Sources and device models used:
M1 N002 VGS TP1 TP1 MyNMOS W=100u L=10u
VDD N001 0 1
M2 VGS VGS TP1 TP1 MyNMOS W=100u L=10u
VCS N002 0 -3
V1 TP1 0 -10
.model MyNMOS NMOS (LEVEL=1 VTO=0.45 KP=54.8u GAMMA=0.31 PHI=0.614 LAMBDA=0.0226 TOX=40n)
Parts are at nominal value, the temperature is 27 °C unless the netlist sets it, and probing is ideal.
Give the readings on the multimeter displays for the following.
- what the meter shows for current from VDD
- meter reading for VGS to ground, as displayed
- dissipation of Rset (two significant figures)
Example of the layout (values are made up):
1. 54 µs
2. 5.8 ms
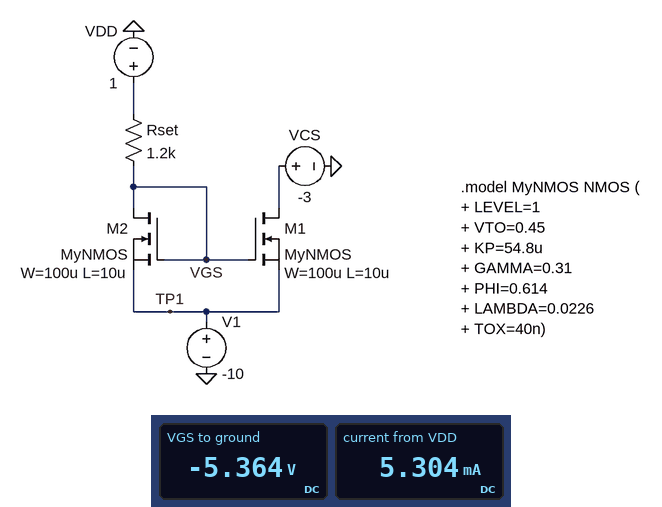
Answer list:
1. 5.304 mA
2. -5.364 V
3. 34 mW
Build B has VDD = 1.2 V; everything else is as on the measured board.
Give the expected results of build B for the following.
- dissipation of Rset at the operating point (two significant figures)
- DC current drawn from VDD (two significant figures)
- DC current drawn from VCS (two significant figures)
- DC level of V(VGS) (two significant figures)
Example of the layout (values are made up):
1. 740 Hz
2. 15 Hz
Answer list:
1. 35 mW
2. 5.4 mA
3. 5.7 mA
4. -5.3 V
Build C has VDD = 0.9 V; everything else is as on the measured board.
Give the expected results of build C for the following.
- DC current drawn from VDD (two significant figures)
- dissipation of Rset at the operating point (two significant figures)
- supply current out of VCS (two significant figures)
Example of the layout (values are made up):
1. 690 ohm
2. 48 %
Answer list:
1. 5.2 mA
2. 33 mW
3. 5.5 mA
